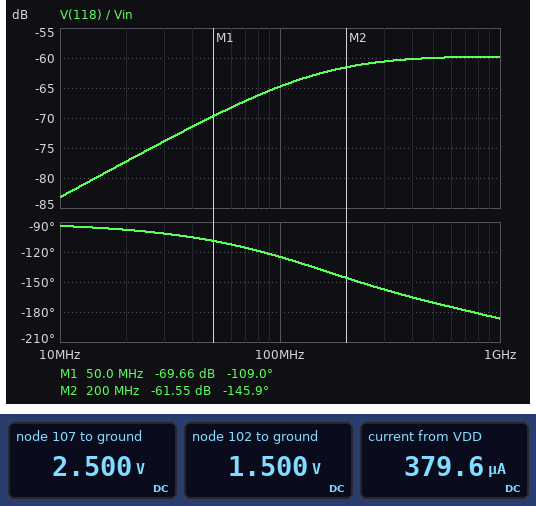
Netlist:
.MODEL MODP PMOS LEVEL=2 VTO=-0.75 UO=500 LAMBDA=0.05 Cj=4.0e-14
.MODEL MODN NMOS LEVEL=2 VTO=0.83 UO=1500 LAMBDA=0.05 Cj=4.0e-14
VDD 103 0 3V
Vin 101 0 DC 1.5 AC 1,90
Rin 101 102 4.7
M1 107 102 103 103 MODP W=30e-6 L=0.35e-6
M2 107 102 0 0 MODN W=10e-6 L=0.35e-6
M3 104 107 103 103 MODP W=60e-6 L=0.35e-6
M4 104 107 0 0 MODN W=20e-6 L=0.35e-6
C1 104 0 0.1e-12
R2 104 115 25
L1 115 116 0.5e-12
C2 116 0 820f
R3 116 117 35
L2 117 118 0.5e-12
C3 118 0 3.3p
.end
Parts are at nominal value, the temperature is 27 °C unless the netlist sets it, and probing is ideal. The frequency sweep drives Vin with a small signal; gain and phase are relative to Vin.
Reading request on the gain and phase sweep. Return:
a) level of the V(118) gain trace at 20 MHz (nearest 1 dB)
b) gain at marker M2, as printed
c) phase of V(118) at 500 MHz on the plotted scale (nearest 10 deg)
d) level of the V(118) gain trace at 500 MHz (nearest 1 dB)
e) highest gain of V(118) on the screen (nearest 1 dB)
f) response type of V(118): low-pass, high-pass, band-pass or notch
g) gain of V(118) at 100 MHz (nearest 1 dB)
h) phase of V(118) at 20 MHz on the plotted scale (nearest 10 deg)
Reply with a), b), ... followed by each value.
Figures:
a) -77 dB
b) -61.55 dB
c) -170 deg
d) -60 dB
e) -60 dB
f) high-pass
g) -65 dB
h) -100 deg
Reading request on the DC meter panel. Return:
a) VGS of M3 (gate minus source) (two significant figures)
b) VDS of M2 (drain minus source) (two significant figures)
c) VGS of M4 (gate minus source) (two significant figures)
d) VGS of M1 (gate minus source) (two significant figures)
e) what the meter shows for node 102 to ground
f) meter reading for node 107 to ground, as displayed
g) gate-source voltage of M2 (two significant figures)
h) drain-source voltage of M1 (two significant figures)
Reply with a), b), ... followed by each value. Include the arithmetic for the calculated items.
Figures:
a) 2.5 V - 3 V = -500 mV
b) 2.5 V = 2.5 V
c) 2.5 V = 2.5 V
d) 1.5 V - 3 V = -1.5 V
e) 1.500 V
f) 2.500 V
g) 1.5 V = 1.5 V
h) 2.5 V - 3 V = -500 mV
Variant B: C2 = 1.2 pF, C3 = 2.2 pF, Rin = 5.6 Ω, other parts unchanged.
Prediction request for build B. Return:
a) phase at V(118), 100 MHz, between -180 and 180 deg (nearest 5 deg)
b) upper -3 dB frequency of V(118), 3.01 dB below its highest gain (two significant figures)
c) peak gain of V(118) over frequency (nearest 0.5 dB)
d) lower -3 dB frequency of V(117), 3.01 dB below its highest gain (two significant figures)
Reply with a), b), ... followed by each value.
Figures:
a) -120 deg
b) 4.9 GHz
c) -58.0 dB
d) 180 MHz
